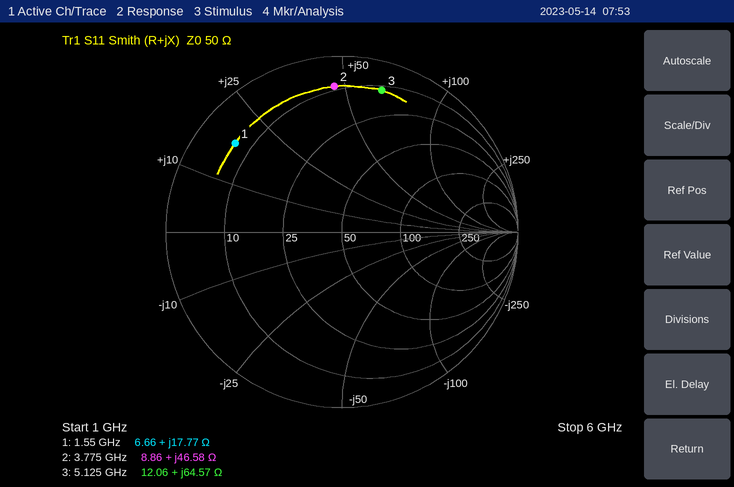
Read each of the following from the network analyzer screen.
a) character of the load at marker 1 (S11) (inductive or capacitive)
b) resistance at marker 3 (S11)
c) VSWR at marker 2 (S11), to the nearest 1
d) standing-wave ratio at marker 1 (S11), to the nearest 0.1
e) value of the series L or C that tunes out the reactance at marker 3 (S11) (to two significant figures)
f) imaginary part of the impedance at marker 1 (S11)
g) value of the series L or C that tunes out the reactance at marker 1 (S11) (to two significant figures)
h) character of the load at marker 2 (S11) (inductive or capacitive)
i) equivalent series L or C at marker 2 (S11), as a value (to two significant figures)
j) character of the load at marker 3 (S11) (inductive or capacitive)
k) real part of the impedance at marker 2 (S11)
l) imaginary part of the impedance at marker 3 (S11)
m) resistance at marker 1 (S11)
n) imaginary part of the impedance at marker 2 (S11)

inductive
12.06 Ω
11
8.5
480 fF
+17.77 Ω
5.8 pF
inductive
2.0 nH
inductive
8.86 Ω
+64.57 Ω
6.66 Ω
+46.58 Ω
